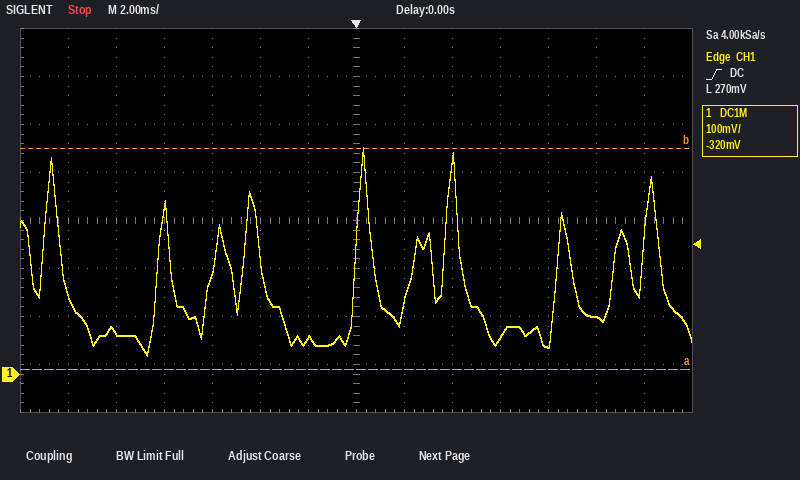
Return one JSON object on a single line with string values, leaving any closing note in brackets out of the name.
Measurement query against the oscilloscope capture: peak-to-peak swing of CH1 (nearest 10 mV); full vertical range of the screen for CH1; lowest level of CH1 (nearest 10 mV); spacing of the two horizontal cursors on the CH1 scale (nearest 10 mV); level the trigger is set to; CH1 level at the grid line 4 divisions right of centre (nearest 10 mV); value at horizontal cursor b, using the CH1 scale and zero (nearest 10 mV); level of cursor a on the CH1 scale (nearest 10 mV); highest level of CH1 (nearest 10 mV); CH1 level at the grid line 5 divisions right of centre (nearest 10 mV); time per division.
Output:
{"peak-to-peak swing of CH1": "430 mV", "full vertical range of the screen for CH1": "800 mV", "lowest level of CH1": "40 mV", "spacing of the two horizontal cursors on the CH1 scale": "460 mV", "level the trigger is set to": "270 mV", "CH1 level at the grid line 4 divisions right of centre": "60 mV", "value at horizontal cursor b, using the CH1 scale and zero": "470 mV", "level of cursor a on the CH1 scale": "10 mV", "highest level of CH1": "470 mV", "CH1 level at the grid line 5 divisions right of centre": "120 mV", "time per division": "2 ms"}
